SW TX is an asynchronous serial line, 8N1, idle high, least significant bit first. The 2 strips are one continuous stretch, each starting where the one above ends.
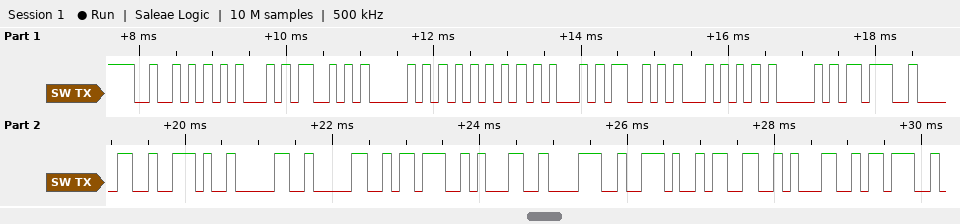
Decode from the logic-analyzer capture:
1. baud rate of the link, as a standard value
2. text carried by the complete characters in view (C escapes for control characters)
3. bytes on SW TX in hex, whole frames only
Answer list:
9600 baud
"RESPUESTA;0.00;18.31;"
52 45 53 50 55 45 53 54 41 3B 30 2E 30 30 3B 31 38 2E 33 31 3B
